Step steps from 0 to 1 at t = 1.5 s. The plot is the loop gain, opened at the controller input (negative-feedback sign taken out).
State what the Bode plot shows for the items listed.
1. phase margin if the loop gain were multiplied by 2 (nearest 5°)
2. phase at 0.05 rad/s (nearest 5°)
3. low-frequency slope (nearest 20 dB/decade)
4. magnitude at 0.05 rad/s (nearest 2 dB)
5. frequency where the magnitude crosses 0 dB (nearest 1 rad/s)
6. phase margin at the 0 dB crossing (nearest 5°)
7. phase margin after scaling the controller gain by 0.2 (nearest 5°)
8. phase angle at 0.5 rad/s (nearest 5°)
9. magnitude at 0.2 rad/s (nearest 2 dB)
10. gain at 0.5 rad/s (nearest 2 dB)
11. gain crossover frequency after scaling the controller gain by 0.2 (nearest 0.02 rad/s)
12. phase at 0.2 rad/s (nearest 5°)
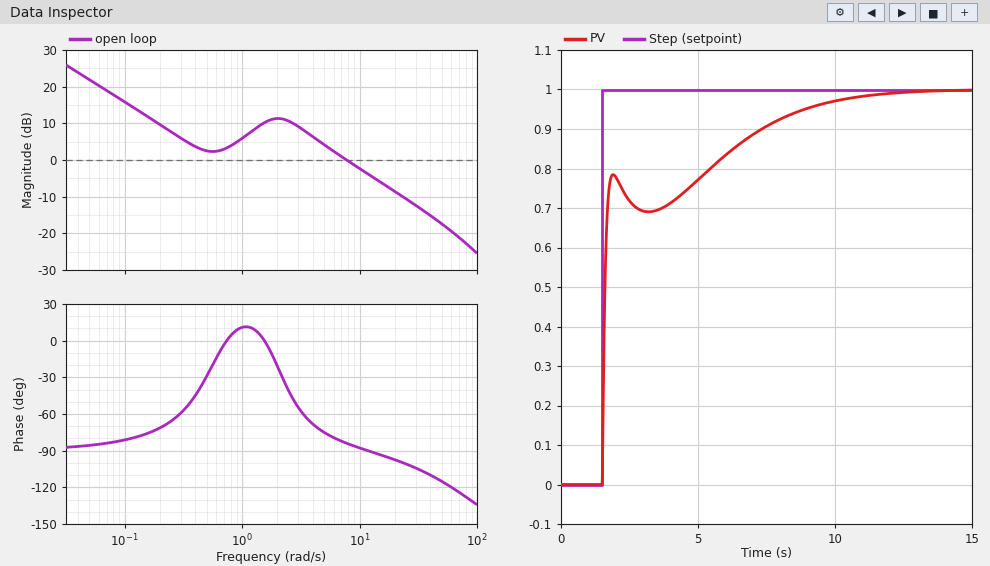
85°
-85°
-20 dB/decade
22 dB
8 rad/s
95°
100°
-30°
10 dB
2 dB
0.12 rad/s
-70°
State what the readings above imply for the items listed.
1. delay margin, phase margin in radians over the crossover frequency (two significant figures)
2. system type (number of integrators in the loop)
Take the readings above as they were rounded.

0.21 s
1
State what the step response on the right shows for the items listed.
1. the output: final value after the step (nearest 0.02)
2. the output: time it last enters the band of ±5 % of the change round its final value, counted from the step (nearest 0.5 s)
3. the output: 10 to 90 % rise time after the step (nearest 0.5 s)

1.00
7.5 s
6.0 s
